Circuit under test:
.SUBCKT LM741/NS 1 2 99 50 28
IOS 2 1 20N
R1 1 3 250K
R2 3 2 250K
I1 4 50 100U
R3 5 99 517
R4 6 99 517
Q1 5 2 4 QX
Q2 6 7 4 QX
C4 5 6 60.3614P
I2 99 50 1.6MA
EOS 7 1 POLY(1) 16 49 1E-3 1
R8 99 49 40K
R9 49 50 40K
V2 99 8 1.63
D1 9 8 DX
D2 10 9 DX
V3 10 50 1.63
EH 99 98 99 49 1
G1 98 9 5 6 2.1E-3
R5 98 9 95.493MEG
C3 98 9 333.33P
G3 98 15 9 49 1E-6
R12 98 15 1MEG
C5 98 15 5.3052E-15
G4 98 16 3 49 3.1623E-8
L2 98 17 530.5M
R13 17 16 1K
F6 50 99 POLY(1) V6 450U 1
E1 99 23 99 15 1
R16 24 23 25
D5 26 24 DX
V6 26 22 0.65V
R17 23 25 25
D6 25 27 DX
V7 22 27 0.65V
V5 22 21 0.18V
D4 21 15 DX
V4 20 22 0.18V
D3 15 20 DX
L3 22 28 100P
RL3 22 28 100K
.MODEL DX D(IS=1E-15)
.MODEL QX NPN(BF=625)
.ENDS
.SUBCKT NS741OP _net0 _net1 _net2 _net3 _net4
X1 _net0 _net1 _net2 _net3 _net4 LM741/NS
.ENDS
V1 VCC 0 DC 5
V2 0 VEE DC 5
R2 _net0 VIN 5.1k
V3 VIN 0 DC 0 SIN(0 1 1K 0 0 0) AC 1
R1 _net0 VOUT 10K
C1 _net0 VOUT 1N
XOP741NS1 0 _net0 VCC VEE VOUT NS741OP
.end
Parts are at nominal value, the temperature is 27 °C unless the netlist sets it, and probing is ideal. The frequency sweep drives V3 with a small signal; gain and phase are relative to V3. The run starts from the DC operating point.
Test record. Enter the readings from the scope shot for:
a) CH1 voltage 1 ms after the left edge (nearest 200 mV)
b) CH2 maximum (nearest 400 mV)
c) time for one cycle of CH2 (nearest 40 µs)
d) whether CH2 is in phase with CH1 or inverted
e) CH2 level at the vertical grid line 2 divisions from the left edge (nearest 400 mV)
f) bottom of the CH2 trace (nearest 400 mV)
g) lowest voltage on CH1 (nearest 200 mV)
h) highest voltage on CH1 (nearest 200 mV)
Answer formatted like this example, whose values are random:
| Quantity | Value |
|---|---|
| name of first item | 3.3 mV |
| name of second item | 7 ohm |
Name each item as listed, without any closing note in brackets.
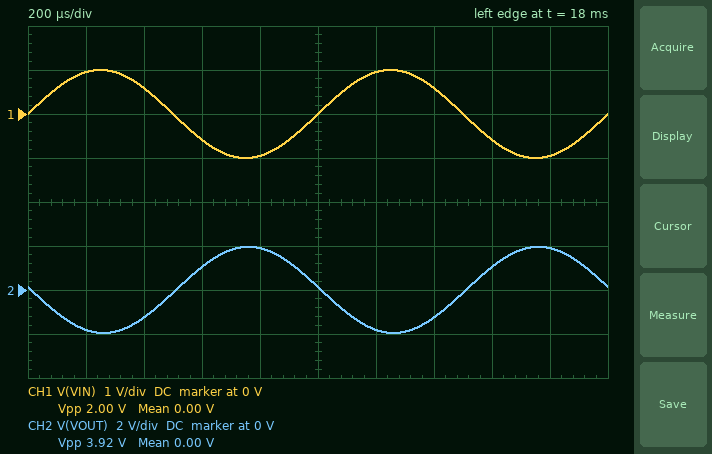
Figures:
| Quantity | Value |
|---|---|
| CH1 voltage 1 ms after the left edge | 0 V |
| CH2 maximum | 2.0 V |
| time for one cycle of CH2 | 1.00 ms |
| whether CH2 is in phase with CH1 or inverted | inverted |
| CH2 level at the vertical grid line 2 divisions from the left edge | -1.2 V |
| bottom of the CH2 trace | -2.0 V |
| lowest voltage on CH1 | -1.0 V |
| highest voltage on CH1 | 1.0 V |
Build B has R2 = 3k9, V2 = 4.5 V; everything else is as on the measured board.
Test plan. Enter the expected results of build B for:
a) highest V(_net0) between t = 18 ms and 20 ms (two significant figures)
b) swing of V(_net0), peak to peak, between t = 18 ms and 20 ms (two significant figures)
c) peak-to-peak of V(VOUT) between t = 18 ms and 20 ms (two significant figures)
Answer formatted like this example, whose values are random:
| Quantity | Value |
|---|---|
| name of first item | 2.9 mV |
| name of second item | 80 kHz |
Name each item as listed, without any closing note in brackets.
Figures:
| Quantity | Value |
|---|---|
| highest V(_net0) between t = 18 ms and 20 ms | 3.6 mV |
| swing of V(_net0), peak to peak, between t = 18 ms and 20 ms | 5.2 mV |
| peak-to-peak of V(VOUT) between t = 18 ms and 20 ms | 5.1 V |
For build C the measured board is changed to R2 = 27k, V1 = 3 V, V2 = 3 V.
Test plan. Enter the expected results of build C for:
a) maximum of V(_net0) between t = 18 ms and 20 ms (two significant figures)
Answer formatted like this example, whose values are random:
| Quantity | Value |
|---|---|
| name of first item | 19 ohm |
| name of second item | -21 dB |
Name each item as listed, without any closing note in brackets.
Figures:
| Quantity | Value |
|---|---|
| maximum of V(_net0) between t = 18 ms and 20 ms | 1.4 mV |
